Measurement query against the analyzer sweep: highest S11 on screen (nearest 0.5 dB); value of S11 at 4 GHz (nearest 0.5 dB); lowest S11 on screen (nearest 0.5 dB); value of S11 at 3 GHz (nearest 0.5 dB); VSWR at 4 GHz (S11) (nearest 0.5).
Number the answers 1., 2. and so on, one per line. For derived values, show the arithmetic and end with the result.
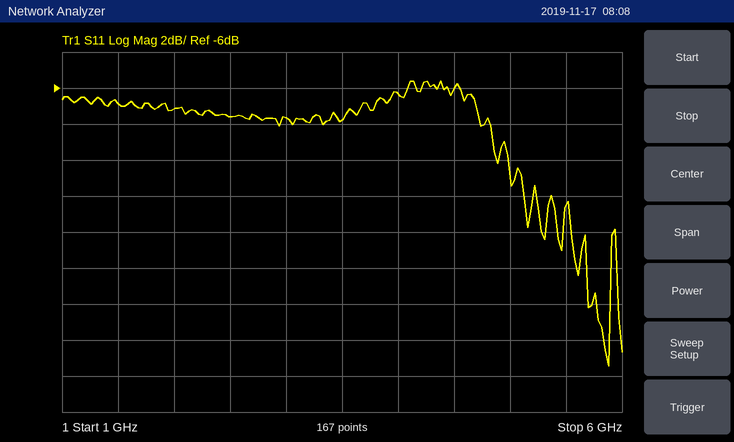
1. -5.5 dB
2. -6.5 dB
3. -21.5 dB
4. -7.5 dB
5. |Γ| = 10^(-6.5/20) = 0.4732; VSWR = (1 + 0.4732)/(1 − 0.4732) ≈ 2.80, so 3.0 to the nearest 0.5
